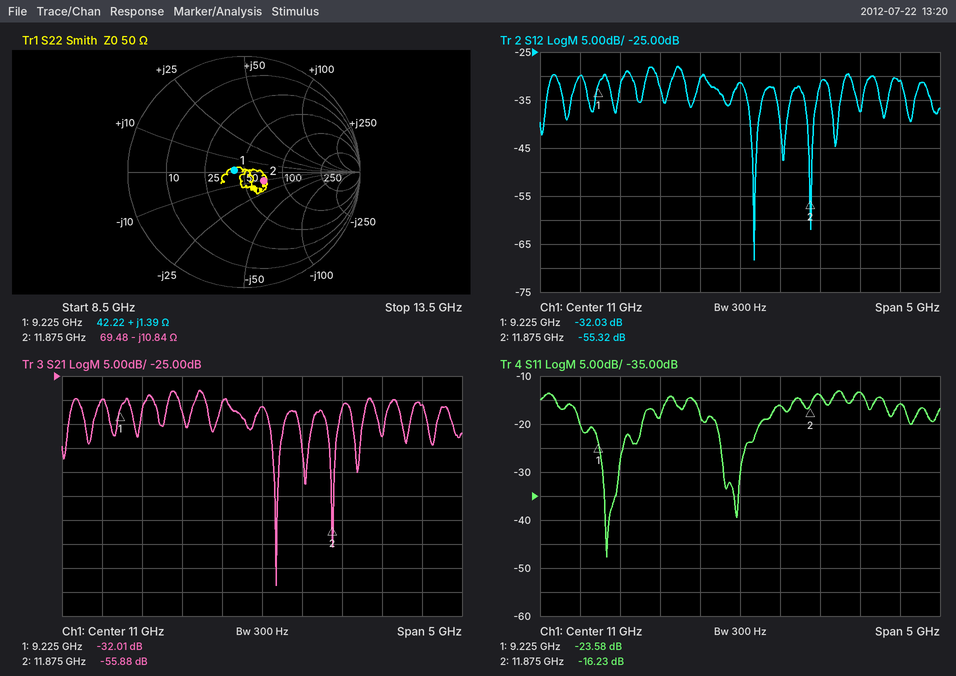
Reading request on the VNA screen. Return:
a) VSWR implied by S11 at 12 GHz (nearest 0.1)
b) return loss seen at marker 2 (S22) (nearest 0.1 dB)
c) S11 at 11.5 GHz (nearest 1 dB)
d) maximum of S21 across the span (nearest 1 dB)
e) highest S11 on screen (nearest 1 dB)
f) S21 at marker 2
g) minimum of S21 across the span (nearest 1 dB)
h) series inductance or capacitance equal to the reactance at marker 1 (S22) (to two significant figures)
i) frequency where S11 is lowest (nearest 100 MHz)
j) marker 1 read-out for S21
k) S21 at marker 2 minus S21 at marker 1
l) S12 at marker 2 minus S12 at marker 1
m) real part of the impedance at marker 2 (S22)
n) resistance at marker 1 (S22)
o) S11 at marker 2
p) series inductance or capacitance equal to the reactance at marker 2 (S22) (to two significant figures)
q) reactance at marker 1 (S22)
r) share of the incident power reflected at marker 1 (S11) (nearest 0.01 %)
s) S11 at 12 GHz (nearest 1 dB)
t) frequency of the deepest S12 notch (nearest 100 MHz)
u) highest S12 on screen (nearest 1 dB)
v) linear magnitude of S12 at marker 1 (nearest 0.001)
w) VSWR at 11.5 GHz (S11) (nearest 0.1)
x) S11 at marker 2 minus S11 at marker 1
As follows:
1.5
14.6 dB
-16 dB
-28 dB
-13 dB
-55.88 dB
-69 dB
24 pH
9.3 GHz
-32.01 dB
-23.87 dB
-23.29 dB
69.48 Ω
42.22 Ω
-16.23 dB
1.2 pF
+1.39 Ω
0.44 %
-14 dB
11.2 GHz
-28 dB
0.025
1.4
7.35 dB
